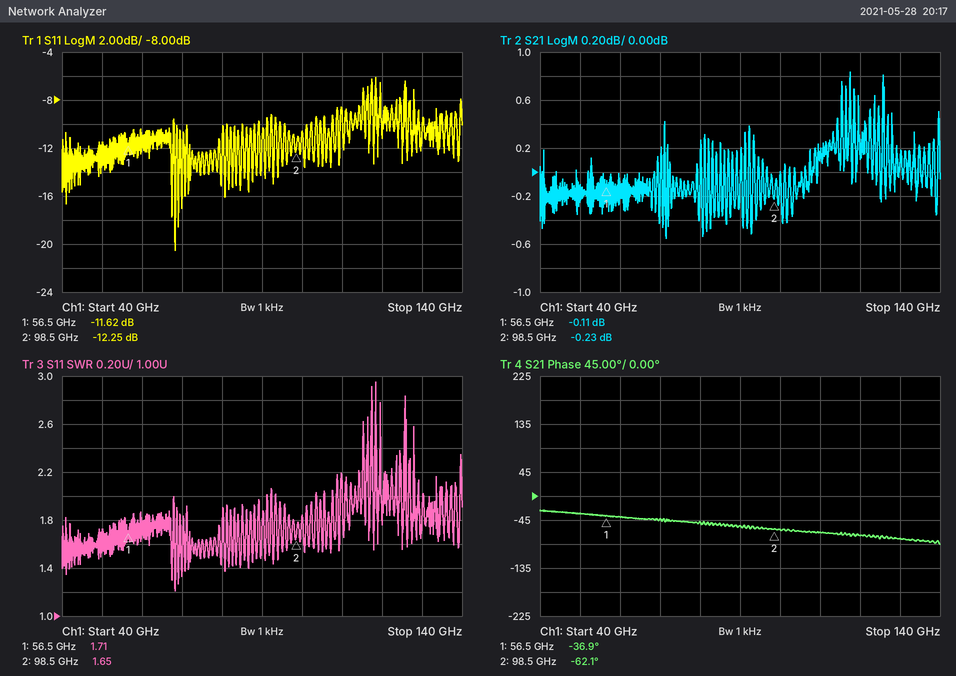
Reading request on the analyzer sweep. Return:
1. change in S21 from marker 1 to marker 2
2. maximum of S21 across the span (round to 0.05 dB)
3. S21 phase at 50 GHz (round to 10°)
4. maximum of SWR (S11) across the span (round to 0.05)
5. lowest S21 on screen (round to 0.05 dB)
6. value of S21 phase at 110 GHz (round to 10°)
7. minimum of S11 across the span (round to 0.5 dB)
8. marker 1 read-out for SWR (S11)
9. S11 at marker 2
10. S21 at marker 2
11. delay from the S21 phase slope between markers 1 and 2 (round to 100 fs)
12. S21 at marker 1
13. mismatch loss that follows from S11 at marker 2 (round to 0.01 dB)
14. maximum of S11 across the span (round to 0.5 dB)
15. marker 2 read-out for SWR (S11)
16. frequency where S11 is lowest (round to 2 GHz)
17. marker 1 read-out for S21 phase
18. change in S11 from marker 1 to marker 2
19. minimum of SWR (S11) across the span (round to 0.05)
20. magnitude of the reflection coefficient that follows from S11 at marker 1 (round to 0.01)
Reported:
-0.12 dB
0.85 dB
-30°
2.95
-0.55 dB
-70°
-20.5 dB
1.71
-12.25 dB
-0.23 dB
1.7 ps
-0.11 dB
0.27 dB
-6.0 dB
1.65
68 GHz
-36.9°
-0.63 dB
1.20
0.26
